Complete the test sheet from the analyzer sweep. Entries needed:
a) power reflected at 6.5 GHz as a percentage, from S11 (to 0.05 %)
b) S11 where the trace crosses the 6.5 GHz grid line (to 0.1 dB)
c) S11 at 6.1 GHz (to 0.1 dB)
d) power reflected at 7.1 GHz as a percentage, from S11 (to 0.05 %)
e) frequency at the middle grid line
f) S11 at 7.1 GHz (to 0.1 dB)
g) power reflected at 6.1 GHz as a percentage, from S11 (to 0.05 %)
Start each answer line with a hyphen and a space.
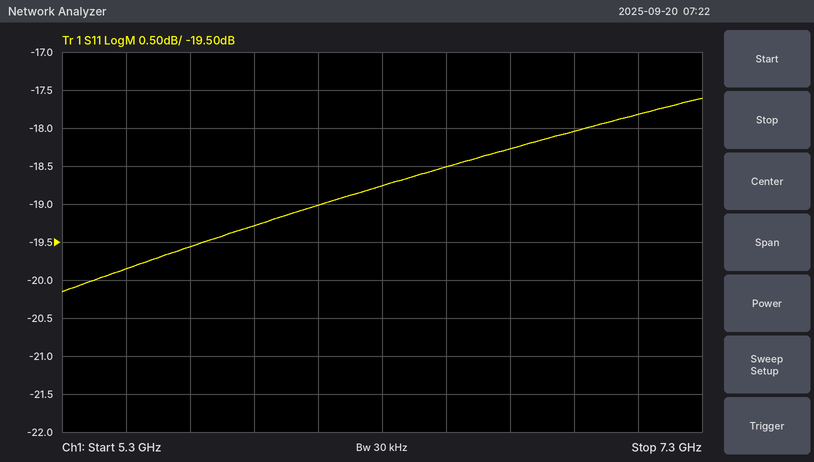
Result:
- 1.40 %
- -18.5 dB
- -19.0 dB
- 1.65 %
- 6.3 GHz
- -17.8 dB
- 1.25 %
